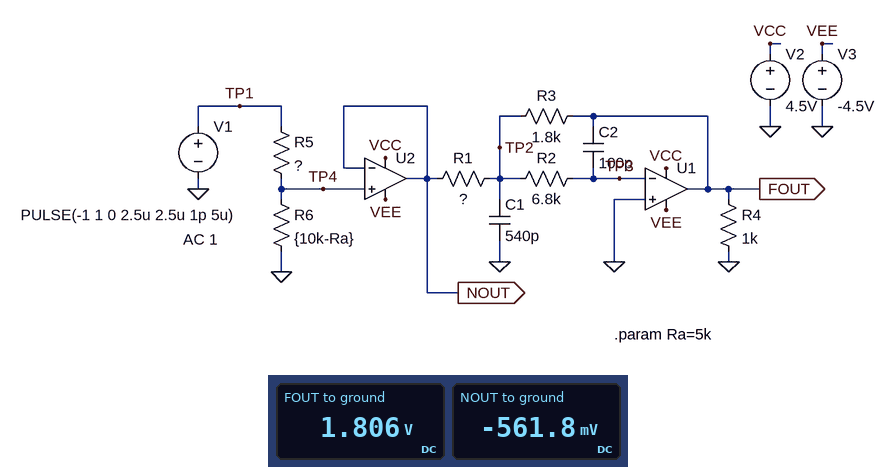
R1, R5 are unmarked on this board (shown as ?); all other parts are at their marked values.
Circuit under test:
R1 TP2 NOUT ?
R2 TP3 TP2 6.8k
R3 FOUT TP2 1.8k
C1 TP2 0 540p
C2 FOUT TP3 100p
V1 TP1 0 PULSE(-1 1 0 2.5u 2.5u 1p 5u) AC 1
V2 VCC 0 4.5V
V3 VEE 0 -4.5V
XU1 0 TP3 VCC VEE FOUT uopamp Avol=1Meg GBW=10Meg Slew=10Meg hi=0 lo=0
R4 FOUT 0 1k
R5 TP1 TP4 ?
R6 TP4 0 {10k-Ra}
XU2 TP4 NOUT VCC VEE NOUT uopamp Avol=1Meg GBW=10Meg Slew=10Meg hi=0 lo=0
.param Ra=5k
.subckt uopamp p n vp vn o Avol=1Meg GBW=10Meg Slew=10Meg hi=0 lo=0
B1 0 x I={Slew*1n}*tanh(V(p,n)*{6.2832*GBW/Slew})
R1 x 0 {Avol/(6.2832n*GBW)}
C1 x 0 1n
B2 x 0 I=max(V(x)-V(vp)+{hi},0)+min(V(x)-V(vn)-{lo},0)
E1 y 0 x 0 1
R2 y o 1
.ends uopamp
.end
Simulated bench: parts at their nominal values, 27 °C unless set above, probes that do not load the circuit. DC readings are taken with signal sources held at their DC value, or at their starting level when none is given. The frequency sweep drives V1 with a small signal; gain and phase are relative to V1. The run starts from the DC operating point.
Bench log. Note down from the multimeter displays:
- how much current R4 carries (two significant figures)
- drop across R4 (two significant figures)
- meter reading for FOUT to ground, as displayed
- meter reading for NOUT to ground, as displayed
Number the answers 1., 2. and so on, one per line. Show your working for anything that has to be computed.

1. (1.806 V) / 1 kΩ = 1.8 mA
2. 1.806 V = 1.8 V
3. 1.806 V
4. -561.8 mV
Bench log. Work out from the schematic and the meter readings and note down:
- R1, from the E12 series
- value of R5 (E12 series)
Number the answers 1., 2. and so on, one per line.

1. 560 Ω
2. 3.9 kΩ
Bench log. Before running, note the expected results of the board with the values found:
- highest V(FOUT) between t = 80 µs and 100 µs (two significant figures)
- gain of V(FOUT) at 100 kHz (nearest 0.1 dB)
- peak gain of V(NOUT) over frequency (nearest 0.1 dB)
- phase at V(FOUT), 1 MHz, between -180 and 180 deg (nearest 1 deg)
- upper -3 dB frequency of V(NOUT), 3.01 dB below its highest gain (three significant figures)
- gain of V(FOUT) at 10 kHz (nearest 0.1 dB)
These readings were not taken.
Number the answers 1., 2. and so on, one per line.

1. 370 mV
2. -1.2 dB
3. -5.0 dB
4. 26 deg
5. 9.98 MHz
6. 5.0 dB
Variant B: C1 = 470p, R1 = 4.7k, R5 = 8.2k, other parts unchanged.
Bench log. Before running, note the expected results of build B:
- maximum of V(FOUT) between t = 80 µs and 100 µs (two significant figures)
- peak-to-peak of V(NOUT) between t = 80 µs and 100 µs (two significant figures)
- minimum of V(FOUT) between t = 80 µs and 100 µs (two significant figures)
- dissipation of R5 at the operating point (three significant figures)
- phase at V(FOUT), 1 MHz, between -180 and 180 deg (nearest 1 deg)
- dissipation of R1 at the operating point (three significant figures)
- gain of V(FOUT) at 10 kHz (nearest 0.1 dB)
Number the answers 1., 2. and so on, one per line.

1. 82 mV
2. 750 mV
3. -82 mV
4. 47.1 µW
5. 6 deg
6. 30.5 µW
7. -16.8 dB
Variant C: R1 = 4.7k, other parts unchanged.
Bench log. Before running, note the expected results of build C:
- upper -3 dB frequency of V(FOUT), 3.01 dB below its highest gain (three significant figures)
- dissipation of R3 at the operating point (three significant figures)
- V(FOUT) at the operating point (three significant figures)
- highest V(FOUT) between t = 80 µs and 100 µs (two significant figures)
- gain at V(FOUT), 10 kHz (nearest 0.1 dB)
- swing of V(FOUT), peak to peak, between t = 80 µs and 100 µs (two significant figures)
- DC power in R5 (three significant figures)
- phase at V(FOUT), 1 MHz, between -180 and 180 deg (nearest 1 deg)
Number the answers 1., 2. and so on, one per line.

1. 199 kHz
2. 25.7 µW
3. 215 mV
4. 120 mV
5. -13.3 dB
6. 240 mV
7. 49.2 µW
8. 4 deg
